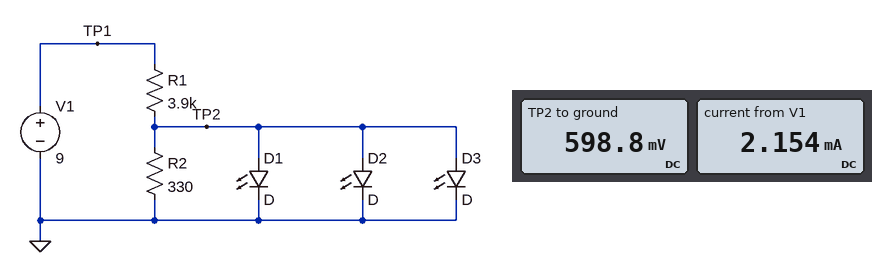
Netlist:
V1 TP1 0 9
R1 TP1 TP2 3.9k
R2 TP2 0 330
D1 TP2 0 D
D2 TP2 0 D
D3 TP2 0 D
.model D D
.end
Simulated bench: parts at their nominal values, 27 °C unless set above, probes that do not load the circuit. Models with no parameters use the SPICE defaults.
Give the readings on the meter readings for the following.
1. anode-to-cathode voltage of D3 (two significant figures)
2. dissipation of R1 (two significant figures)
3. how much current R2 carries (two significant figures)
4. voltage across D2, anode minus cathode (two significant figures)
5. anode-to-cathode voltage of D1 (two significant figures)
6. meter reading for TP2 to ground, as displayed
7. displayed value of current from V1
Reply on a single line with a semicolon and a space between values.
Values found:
600 mV; 18 mW; 1.8 mA; 600 mV; 600 mV; 598.8 mV; 2.154 mA
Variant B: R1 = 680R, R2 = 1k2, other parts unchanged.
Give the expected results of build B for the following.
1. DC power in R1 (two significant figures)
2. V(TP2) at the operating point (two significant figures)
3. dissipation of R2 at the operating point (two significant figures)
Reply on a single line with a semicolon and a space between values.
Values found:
100 mW; 690 mV; 400 µW
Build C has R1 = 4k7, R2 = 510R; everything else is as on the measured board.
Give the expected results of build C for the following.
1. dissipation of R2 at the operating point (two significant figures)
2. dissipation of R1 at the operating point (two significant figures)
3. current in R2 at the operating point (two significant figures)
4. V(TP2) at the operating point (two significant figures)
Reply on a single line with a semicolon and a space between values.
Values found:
740 µW; 15 mW; 1.2 mA; 610 mV
